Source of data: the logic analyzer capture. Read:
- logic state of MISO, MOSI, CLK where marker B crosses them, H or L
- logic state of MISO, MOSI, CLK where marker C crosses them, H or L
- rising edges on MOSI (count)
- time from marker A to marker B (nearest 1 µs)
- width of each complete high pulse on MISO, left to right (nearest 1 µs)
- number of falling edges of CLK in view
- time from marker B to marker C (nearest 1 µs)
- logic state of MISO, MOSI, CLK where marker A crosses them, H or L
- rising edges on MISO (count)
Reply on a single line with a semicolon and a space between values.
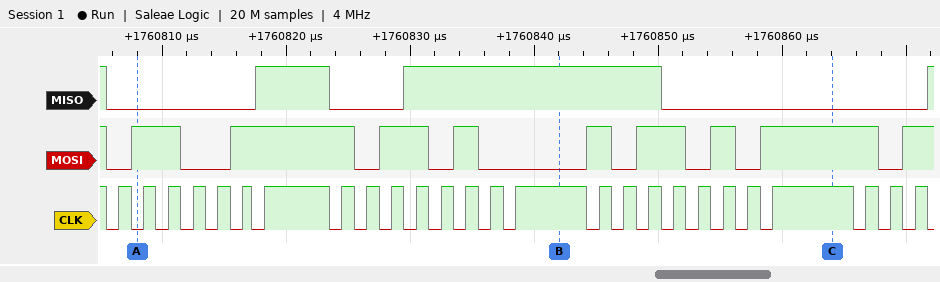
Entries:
MISO=H, MOSI=L, CLK=H; MISO=L, MOSI=H, CLK=H; 9; 34 µs; 6 µs, 21 µs; 27; 22 µs; MISO=L, MOSI=H, CLK=L; 3
